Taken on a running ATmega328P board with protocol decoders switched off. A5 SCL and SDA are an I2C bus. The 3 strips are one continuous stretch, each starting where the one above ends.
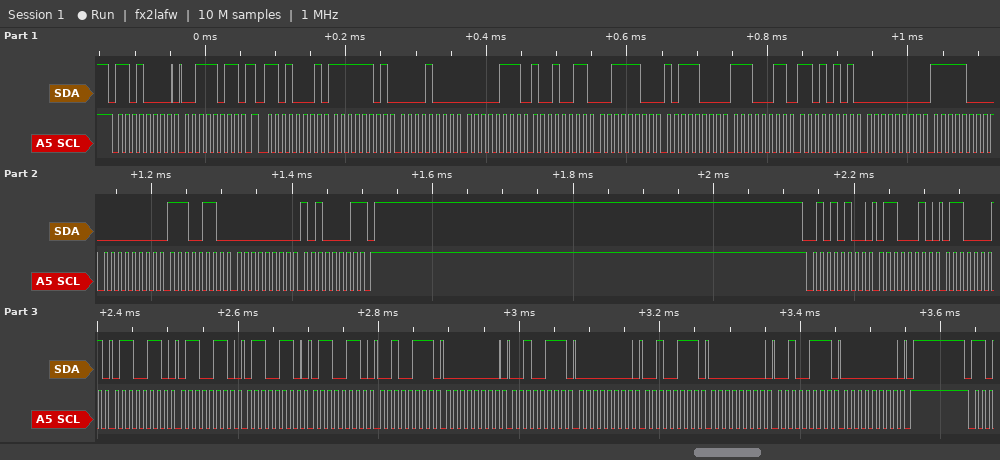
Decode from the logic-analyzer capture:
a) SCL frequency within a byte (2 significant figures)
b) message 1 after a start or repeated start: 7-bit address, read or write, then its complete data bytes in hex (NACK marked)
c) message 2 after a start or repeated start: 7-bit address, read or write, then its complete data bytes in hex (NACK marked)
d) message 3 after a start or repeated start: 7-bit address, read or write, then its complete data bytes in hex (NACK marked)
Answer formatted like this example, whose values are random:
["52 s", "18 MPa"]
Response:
["100 kHz", "0x68 write: 3B", "0x68 read: FD 08 07 93 3C B8 E3 D5 00 F8 00 E6 00 A1 NACK", "0x2A write: 62 61 66 66 66 66 27 00 27 00 27 00 27 00"]
